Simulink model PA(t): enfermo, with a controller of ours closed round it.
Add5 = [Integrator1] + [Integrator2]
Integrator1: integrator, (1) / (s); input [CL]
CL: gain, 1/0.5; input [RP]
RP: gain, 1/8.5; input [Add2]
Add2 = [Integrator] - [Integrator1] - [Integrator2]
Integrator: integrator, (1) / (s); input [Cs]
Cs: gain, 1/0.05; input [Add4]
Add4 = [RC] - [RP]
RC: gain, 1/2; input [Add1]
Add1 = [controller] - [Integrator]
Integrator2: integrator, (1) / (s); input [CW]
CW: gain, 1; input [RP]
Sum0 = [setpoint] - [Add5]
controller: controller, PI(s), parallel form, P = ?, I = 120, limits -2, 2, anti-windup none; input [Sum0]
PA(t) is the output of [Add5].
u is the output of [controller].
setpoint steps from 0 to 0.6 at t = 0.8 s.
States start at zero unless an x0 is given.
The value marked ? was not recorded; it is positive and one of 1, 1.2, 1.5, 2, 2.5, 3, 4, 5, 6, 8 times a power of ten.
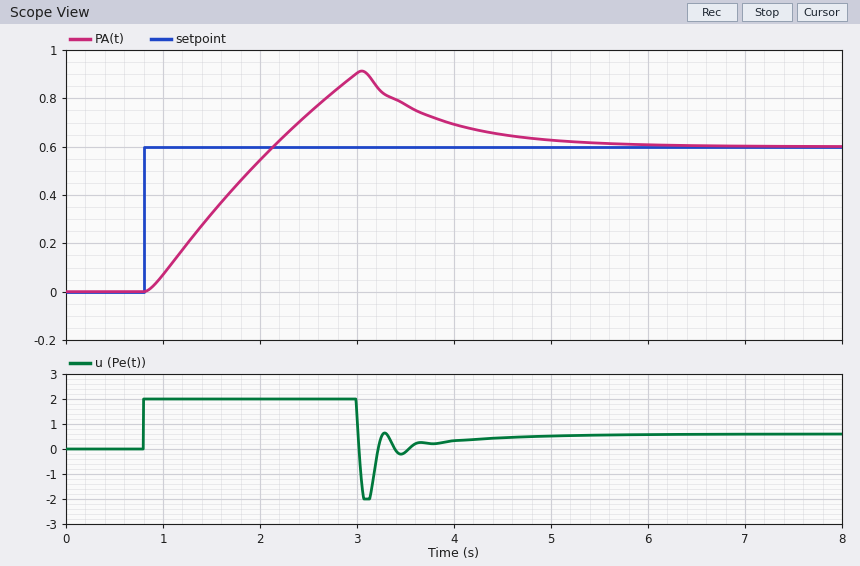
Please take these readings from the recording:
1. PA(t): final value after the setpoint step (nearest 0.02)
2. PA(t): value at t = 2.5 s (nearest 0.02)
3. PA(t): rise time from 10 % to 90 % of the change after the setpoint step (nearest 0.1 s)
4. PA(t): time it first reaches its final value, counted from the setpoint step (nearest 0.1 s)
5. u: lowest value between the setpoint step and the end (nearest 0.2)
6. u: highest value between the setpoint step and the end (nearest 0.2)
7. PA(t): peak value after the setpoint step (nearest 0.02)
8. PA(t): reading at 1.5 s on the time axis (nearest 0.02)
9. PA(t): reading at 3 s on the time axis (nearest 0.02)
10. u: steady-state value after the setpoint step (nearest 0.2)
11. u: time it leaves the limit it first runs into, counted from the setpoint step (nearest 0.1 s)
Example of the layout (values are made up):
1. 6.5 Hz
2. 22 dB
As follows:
1. 0.60
2. 0.74
3. 1.0 s
4. 1.3 s
5. -2.0
6. 2.0
7. 0.92
8. 0.32
9. 0.90
10. 0.6
11. 2.2 s
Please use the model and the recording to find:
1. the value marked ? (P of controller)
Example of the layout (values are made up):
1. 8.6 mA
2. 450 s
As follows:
1. 100
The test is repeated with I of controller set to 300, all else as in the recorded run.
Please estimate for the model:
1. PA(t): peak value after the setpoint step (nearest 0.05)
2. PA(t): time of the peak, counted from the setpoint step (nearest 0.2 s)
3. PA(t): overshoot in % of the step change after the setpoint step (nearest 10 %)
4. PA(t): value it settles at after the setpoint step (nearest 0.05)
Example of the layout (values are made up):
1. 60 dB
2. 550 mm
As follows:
1. 1.00
2. 2.6 s
3. 70 %
4. 0.60
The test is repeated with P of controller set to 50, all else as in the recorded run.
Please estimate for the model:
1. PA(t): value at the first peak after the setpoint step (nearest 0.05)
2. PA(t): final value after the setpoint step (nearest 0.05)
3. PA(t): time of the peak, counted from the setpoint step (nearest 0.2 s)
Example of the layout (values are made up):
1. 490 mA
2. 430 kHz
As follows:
1. 1.00
2. 0.60
3. 2.6 s
